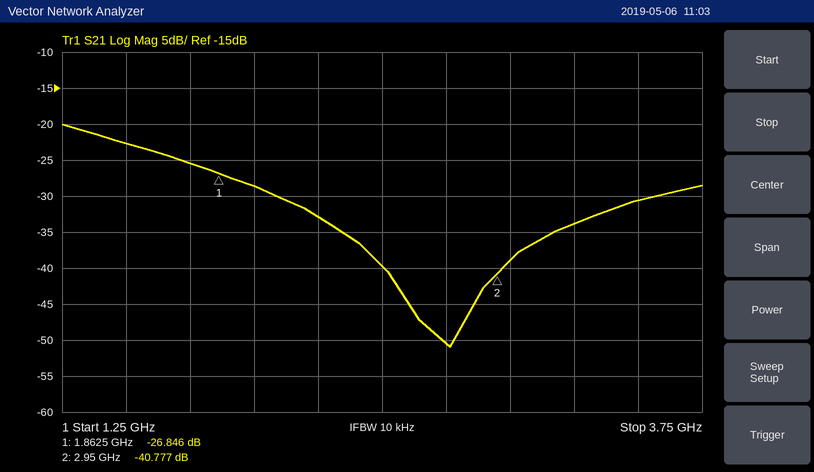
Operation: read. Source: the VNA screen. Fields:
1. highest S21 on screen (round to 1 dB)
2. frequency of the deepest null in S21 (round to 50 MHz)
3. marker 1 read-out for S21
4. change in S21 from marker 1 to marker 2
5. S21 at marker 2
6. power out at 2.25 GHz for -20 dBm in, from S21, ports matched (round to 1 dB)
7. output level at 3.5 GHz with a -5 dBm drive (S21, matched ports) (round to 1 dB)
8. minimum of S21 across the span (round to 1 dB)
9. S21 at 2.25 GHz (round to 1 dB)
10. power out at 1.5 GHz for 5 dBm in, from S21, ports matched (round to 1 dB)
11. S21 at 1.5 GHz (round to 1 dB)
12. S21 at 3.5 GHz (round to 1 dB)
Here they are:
-20 dB
2.75 GHz
-26.846 dB
-13.931 dB
-40.777 dB
-53 dBm
-36 dBm
-51 dB
-33 dB
-18 dBm
-23 dB
-31 dB
